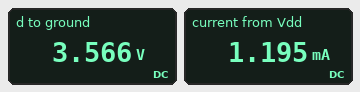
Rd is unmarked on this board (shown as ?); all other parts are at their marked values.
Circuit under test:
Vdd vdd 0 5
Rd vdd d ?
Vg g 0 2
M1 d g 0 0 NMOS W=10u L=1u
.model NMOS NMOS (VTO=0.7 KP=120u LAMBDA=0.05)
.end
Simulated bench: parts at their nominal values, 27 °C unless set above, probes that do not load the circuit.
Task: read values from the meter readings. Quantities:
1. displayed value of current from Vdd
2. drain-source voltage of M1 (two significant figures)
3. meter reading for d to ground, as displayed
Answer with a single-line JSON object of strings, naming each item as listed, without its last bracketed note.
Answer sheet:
{"displayed value of current from Vdd": "1.195 mA", "drain-source voltage of M1": "3.6 V", "meter reading for d to ground, as displayed": "3.566 V"}
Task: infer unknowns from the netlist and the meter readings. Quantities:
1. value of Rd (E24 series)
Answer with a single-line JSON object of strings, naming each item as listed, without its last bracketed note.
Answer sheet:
{"value of Rd": "1.2 kΩ"}
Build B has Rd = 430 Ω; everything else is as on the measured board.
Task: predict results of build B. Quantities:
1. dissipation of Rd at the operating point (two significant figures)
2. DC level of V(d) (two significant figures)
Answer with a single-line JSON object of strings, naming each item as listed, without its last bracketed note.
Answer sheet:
{"dissipation of Rd at the operating point": "660 µW", "DC level of V(d)": "4.5 V"}
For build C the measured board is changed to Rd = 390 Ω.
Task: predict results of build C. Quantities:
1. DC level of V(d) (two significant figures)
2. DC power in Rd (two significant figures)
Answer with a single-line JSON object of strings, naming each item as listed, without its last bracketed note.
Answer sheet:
{"DC level of V(d)": "4.5 V", "DC power in Rd": "600 µW"}
